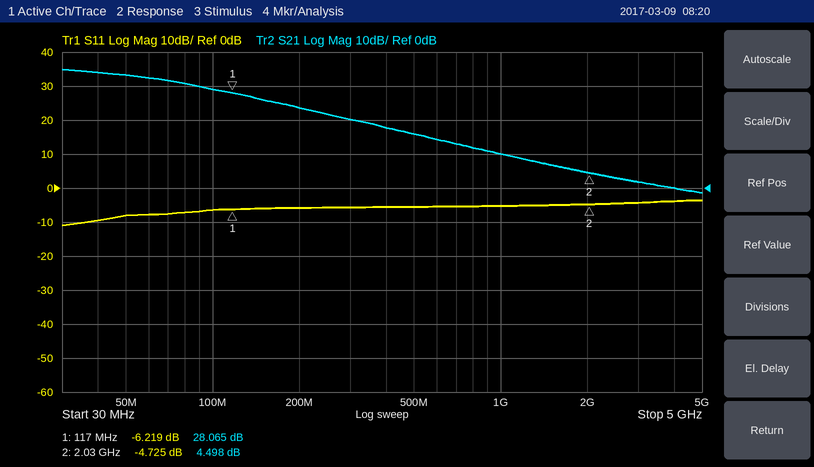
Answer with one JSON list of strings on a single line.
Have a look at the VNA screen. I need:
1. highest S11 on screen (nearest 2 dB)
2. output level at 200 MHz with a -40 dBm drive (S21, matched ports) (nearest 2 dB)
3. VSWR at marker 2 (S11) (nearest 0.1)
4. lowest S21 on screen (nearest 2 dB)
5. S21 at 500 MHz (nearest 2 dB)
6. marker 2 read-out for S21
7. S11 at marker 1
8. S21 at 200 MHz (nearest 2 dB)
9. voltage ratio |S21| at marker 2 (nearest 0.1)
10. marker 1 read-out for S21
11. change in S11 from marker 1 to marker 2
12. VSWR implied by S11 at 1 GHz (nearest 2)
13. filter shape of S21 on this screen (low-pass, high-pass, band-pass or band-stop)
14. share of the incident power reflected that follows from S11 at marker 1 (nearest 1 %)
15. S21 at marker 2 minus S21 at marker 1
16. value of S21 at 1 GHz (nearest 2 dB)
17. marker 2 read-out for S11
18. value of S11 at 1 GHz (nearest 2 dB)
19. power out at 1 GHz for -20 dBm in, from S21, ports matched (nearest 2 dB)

["-4 dB", "-16 dBm", "3.8", "-2 dB", "16 dB", "4.498 dB", "-6.219 dB", "24 dB", "1.7", "28.065 dB", "1.494 dB", "4", "low-pass", "24 %", "-23.567 dB", "10 dB", "-4.725 dB", "-6 dB", "-10 dBm"]
